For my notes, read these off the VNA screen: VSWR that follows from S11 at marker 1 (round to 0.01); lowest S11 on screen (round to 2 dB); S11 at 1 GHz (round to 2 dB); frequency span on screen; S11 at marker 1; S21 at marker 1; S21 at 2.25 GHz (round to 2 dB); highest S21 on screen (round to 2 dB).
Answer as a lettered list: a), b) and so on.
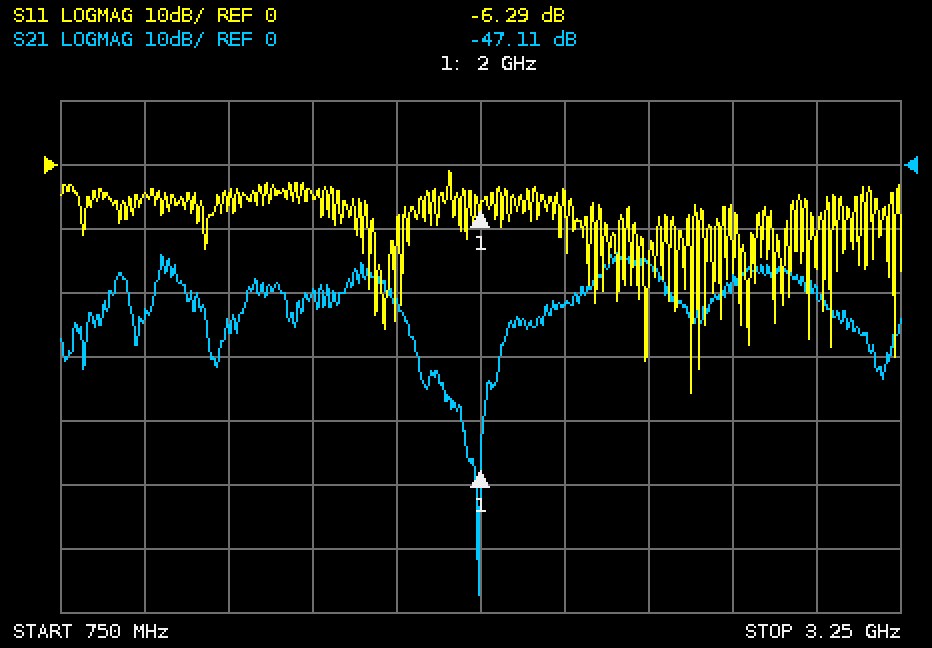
a) 2.88
b) -36 dB
c) -4 dB
d) 2.5 GHz
e) -6.29 dB
f) -47.11 dB
g) -22 dB
h) -14 dB
